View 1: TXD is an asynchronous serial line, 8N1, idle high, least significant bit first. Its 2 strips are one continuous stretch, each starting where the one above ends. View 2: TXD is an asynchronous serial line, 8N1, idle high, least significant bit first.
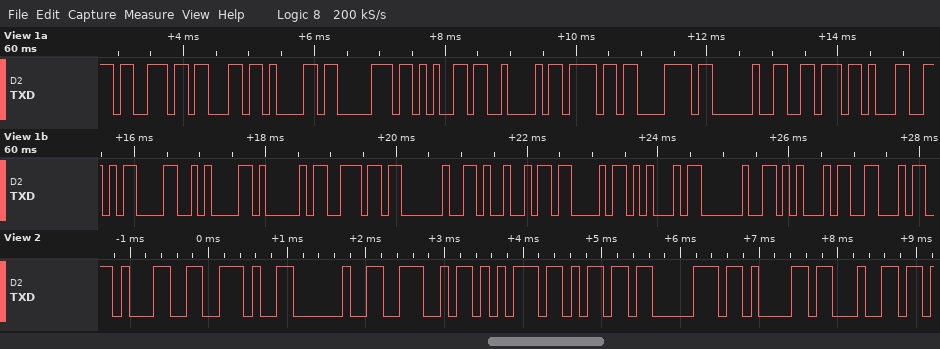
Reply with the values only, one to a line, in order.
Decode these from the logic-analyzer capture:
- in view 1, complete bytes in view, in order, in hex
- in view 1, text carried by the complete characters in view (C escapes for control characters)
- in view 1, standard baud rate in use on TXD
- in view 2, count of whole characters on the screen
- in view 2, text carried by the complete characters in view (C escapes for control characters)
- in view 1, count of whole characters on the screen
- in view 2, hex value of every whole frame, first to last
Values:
0x73 0x63 0x61 0x70 0x65 0x42 0x6F 0x78 0x20 0x76 0x31 0x0D 0x0A 0x41 0x6E 0x20 0x49 0x43 0x45 0x20 0x45 0x46
"scapeBox v1\r\nAn ICE EF"
9600 baud
9
"1. Numpad"
22
31 2E 20 4E 75 6D 70 61 64
